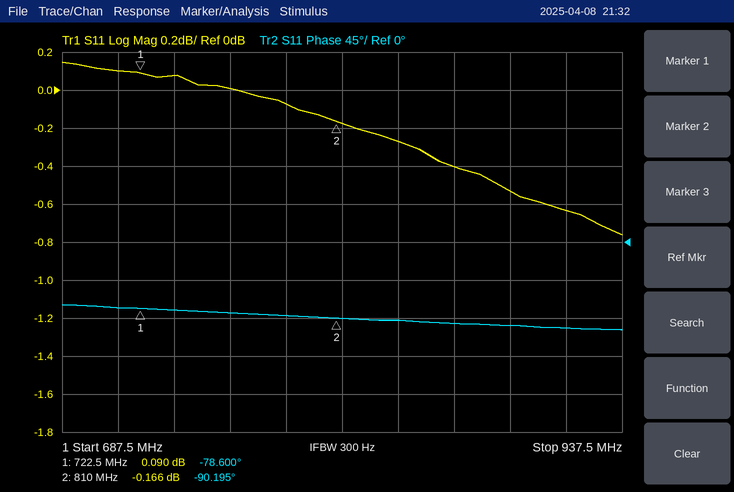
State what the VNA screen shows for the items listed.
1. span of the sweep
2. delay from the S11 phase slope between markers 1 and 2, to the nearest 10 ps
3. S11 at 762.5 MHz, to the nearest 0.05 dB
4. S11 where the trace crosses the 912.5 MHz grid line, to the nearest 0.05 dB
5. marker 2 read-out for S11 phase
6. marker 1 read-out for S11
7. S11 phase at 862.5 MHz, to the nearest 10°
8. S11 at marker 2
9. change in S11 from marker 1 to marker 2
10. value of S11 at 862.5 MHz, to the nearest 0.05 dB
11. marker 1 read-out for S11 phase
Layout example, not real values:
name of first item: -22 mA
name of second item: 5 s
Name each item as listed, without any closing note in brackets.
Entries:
span of the sweep: 250 MHz
delay from the S11 phase slope between markers 1 and 2, to the nearest 10 ps: 370 ps
S11 at 762.5 MHz, to the nearest 0.05 dB: 0.00 dB
S11 where the trace crosses the 912.5 MHz grid line, to the nearest 0.05 dB: -0.65 dB
marker 2 read-out for S11 phase: -90.195°
marker 1 read-out for S11: 0.090 dB
S11 phase at 862.5 MHz, to the nearest 10°: -100°
S11 at marker 2: -0.166 dB
change in S11 from marker 1 to marker 2: -0.256 dB
value of S11 at 862.5 MHz, to the nearest 0.05 dB: -0.40 dB
marker 1 read-out for S11 phase: -78.600°
